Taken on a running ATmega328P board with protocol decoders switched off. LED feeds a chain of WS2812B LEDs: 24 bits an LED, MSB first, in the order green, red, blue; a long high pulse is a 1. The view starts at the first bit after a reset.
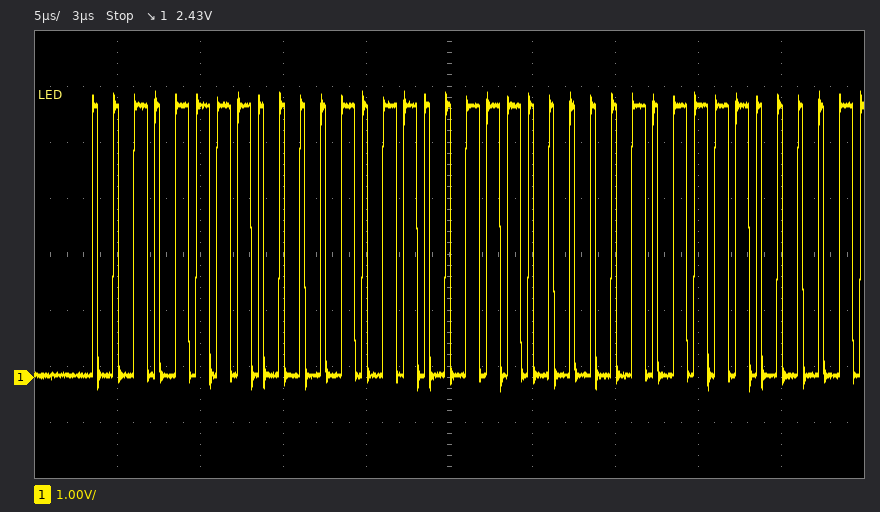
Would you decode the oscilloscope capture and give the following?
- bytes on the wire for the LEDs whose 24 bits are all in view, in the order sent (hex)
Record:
2F 0B 38
